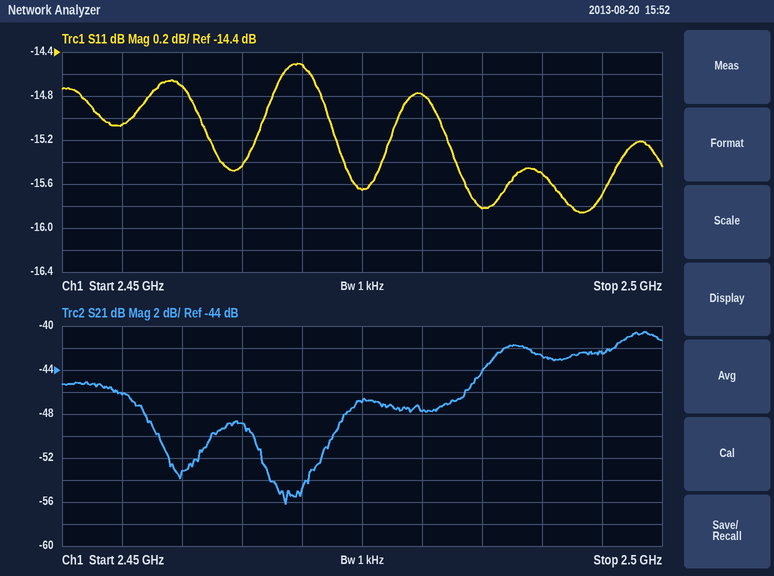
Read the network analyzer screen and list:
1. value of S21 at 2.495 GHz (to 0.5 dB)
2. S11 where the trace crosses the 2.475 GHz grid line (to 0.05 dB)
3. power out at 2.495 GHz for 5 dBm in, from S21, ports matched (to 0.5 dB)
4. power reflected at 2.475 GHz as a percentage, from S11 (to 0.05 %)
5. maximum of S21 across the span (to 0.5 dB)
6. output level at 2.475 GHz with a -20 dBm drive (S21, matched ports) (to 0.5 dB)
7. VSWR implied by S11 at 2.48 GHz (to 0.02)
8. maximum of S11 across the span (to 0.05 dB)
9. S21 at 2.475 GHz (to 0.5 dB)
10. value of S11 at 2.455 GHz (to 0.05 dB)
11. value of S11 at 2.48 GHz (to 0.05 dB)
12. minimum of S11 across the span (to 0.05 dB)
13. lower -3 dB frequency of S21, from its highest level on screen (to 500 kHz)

-42.5 dB
-15.65 dB
-37.5 dBm
2.70 %
-40.5 dB
-67.0 dBm
1.44
-14.50 dB
-47.0 dB
-15.05 dB
-14.80 dB
-15.85 dB
2.4855 GHz
